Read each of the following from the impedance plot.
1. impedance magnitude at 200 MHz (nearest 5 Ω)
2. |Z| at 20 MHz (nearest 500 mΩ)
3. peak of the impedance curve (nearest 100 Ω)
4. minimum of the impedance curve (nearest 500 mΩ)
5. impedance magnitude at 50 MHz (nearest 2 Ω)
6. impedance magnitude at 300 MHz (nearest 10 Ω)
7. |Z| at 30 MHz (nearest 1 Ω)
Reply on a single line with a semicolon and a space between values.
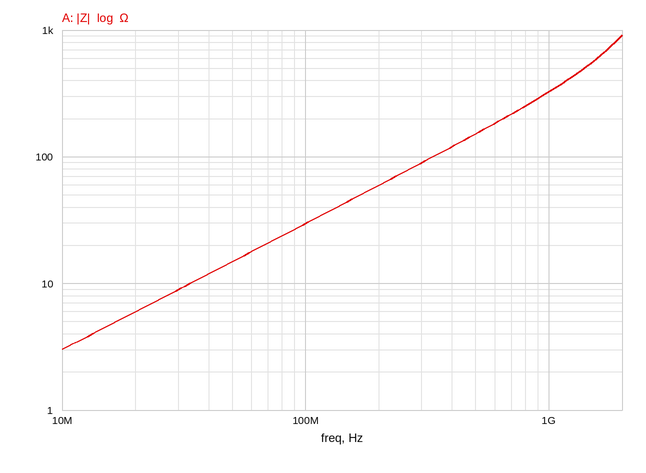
60 Ω; 6.0 Ω; 900 Ω; 3.0 Ω; 14 Ω; 90 Ω; 9 Ω
